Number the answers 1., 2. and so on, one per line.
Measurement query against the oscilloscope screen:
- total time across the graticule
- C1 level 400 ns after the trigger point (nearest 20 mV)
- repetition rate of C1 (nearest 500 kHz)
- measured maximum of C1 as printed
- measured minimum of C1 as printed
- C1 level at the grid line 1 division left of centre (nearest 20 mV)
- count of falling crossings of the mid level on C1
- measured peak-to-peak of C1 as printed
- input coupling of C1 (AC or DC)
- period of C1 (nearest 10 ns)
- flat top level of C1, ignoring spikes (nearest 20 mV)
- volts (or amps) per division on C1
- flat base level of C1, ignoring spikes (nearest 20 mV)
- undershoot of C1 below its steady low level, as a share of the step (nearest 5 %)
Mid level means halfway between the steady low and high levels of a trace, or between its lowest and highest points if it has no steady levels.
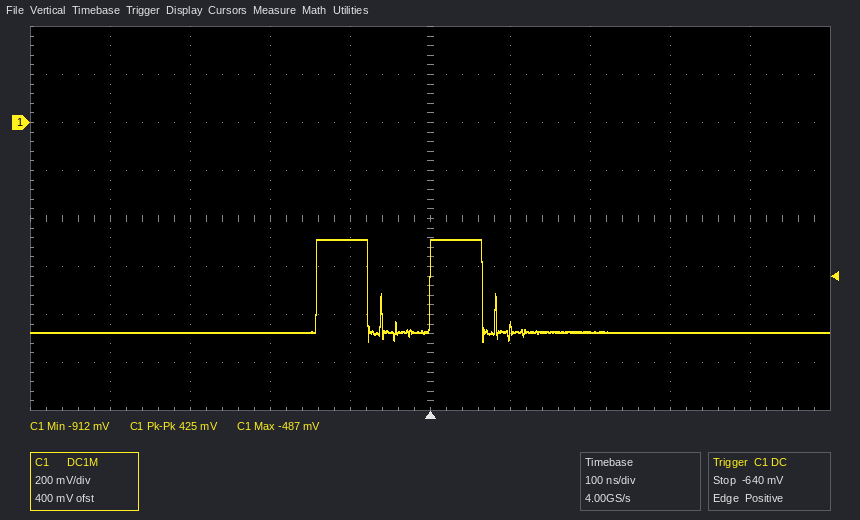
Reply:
1. 1 µs
2. -880 mV
3. 7.0 MHz
4. -487 mV
5. -912 mV
6. -480 mV
7. 2
8. 425 mV
9. DC
10. 140 ns
11. -480 mV
12. 200 mV
13. -880 mV
14. 10 %
